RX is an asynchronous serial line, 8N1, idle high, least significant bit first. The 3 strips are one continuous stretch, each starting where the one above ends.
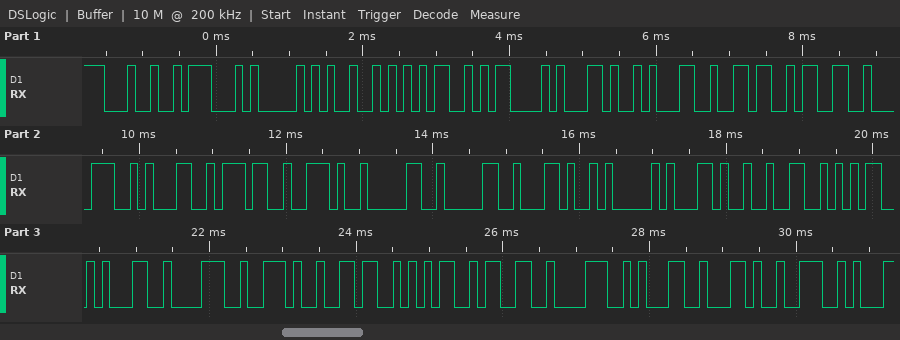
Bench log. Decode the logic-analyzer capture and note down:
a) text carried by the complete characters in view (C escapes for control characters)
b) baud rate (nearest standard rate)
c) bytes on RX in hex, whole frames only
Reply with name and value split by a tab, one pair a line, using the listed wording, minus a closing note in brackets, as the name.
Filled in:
text carried by the complete characters in view	"$GPRMC,163817.00,A,2518.65381,N"
baud rate	9600 baud
bytes on RX in hex, whole frames only	0x24 0x47 0x50 0x52 0x4D 0x43 0x2C 0x31 0x36 0x33 0x38 0x31 0x37 0x2E 0x30 0x30 0x2C 0x41 0x2C 0x32 0x35 0x31 0x38 0x2E 0x36 0x35 0x33 0x38 0x31 0x2C 0x4E
